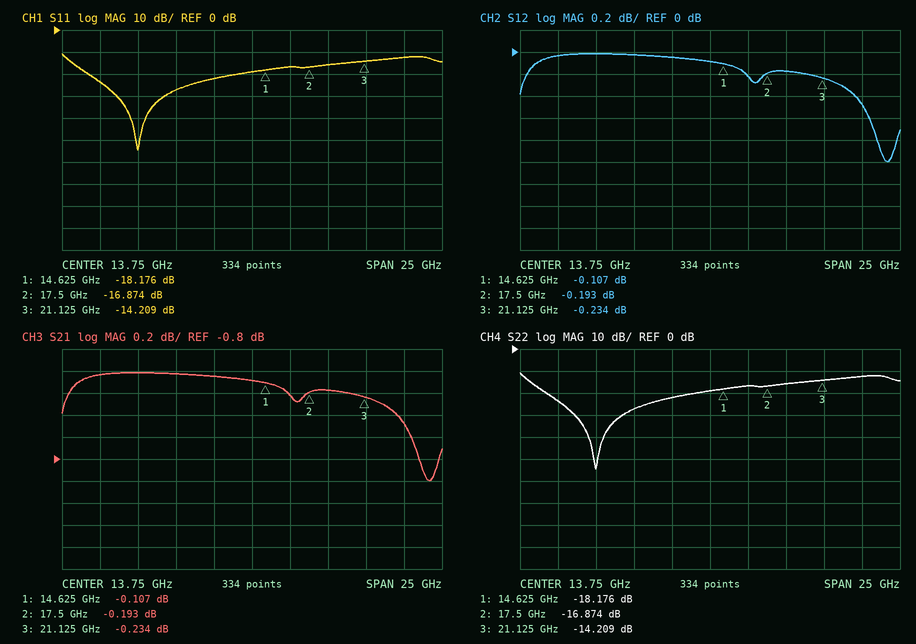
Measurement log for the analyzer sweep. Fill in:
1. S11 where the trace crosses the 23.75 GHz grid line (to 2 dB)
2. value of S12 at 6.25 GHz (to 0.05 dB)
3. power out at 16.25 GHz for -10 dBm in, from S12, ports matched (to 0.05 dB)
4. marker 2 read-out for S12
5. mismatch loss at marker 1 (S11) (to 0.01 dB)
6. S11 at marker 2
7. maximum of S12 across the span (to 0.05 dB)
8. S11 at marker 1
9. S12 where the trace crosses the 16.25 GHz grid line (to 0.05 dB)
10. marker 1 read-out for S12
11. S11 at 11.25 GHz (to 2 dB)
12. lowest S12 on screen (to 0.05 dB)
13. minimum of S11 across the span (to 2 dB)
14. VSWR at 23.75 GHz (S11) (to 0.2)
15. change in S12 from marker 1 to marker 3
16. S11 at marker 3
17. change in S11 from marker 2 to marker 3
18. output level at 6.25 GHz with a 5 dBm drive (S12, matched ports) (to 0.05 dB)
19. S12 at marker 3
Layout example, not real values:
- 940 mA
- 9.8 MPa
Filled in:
- -12 dB
- 0.00 dB
- -10.20 dBm
- -0.193 dB
- 0.07 dB
- -16.874 dB
- 0.00 dB
- -18.176 dB
- -0.20 dB
- -0.107 dB
- -22 dB
- -1.00 dB
- -54 dB
- 1.6
- -0.127 dB
- -14.209 dB
- 2.665 dB
- 5.00 dBm
- -0.234 dB
